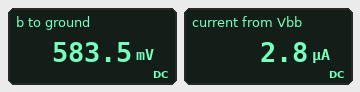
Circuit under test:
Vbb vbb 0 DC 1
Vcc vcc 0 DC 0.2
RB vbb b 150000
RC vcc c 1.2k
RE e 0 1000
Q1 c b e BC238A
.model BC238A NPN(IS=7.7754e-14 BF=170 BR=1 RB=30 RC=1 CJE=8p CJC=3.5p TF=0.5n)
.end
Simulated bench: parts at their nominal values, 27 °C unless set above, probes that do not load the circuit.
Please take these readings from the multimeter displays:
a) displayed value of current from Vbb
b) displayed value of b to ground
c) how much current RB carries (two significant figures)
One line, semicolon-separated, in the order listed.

2.8 µA; 583.5 mV; 2.8 µA
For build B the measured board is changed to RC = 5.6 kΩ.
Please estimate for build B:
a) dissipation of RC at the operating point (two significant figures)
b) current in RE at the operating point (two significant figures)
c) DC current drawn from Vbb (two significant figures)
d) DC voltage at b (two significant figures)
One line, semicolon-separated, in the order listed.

2.5 µW; 24 µA; 3.1 µA; 530 mV
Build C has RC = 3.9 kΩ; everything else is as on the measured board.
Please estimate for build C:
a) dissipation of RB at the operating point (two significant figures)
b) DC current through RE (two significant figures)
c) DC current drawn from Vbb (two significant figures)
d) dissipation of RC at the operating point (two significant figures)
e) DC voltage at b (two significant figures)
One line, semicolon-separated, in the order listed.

1.4 µW; 30 µA; 3.0 µA; 2.9 µW; 540 mV
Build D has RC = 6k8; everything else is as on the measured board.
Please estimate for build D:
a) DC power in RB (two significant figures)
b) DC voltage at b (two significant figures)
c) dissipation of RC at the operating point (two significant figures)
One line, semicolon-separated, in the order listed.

1.5 µW; 530 mV; 2.3 µW
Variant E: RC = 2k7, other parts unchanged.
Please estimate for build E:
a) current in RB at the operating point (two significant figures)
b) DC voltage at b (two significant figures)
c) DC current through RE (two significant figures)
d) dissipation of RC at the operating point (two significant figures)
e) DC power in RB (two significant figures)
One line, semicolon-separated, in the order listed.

3.0 µA; 560 mV; 37 µA; 3.2 µW; 1.3 µW
